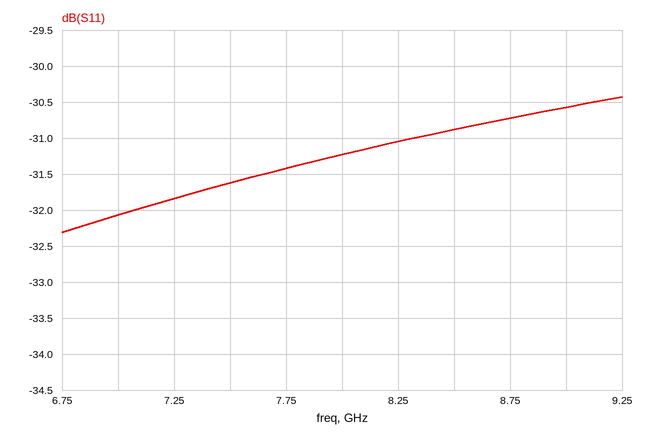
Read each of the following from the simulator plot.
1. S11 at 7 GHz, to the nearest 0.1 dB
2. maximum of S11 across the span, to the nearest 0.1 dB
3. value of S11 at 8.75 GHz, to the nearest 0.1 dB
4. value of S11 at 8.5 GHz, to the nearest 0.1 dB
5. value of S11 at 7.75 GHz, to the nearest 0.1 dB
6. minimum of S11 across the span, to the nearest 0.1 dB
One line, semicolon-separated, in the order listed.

-32.1 dB; -30.4 dB; -30.7 dB; -30.9 dB; -31.4 dB; -32.3 dB
